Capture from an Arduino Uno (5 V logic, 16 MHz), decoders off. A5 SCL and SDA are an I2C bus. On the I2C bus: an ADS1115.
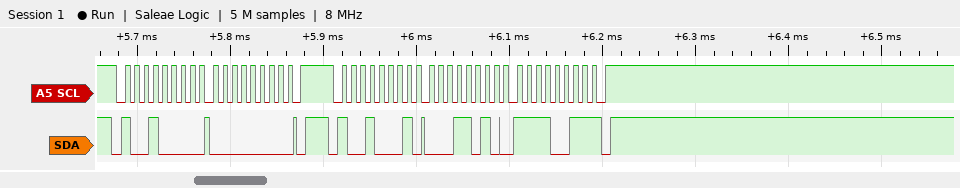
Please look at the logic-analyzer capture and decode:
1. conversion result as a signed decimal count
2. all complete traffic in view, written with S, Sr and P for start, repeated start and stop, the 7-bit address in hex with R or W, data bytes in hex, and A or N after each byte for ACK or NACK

6899
S 48W A 00 A P S 48R A 1A A F3 N P
